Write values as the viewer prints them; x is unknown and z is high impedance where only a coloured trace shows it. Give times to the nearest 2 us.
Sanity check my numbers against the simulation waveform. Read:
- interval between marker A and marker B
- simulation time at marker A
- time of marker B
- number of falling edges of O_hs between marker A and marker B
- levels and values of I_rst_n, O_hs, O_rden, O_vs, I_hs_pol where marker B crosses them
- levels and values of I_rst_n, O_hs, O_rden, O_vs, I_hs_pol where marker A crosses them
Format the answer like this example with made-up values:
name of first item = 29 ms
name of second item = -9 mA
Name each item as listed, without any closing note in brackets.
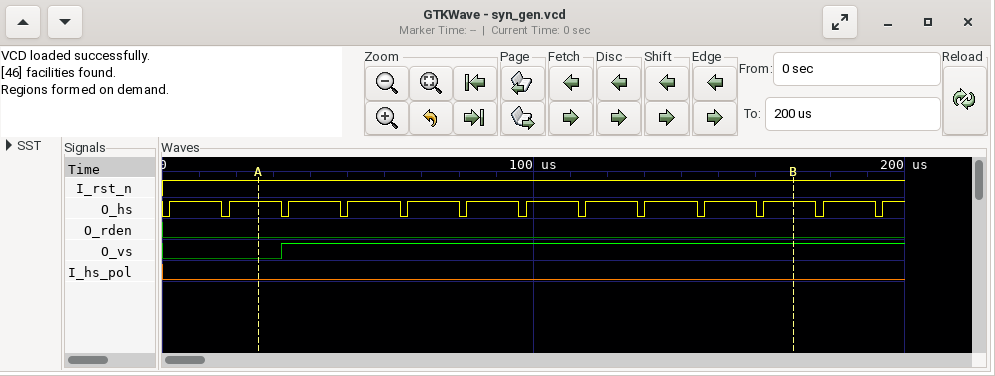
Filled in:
interval between marker A and marker B = 144 us
simulation time at marker A = 26 us
time of marker B = 170 us
number of falling edges of O_hs between marker A and marker B = 9
levels and values of I_rst_n, O_hs, O_rden, O_vs, I_hs_pol where marker B crosses them = I_rst_n=1, O_hs=1, O_rden=0, O_vs=1, I_hs_pol=0
levels and values of I_rst_n, O_hs, O_rden, O_vs, I_hs_pol where marker A crosses them = I_rst_n=1, O_hs=1, O_rden=0, O_vs=0, I_hs_pol=0
